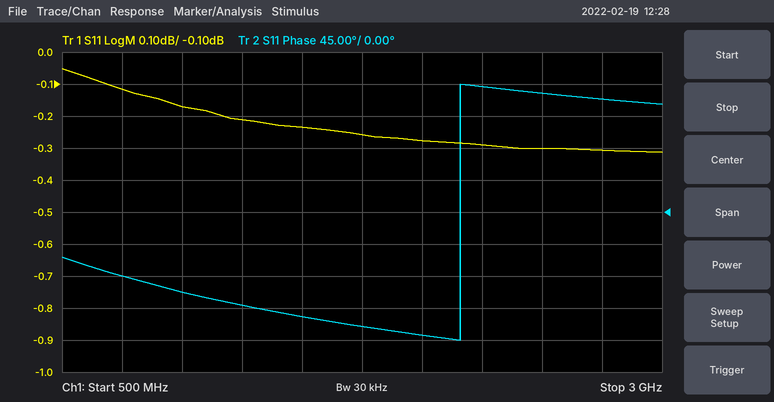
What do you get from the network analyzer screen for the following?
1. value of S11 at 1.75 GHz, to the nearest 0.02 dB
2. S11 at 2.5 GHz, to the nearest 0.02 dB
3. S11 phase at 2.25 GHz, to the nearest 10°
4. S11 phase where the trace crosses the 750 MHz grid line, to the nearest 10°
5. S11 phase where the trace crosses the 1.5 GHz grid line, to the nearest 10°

-0.26 dB
-0.30 dB
180°
-90°
-150°
